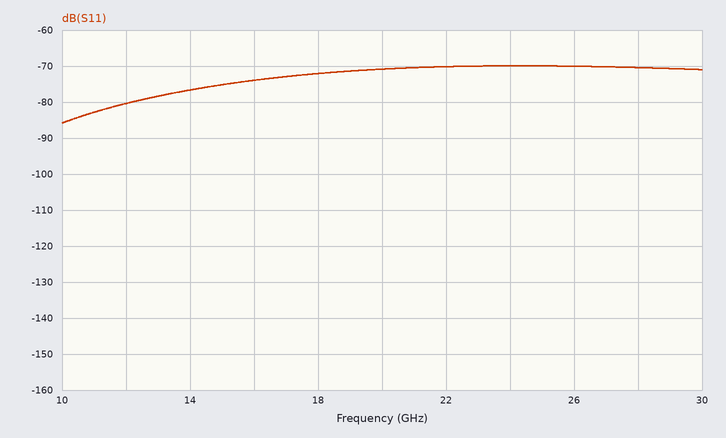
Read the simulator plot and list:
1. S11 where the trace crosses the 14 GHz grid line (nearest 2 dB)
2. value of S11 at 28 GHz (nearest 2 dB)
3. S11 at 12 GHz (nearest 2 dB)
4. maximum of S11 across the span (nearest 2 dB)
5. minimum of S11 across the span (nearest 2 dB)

-76 dB
-70 dB
-80 dB
-70 dB
-86 dB
